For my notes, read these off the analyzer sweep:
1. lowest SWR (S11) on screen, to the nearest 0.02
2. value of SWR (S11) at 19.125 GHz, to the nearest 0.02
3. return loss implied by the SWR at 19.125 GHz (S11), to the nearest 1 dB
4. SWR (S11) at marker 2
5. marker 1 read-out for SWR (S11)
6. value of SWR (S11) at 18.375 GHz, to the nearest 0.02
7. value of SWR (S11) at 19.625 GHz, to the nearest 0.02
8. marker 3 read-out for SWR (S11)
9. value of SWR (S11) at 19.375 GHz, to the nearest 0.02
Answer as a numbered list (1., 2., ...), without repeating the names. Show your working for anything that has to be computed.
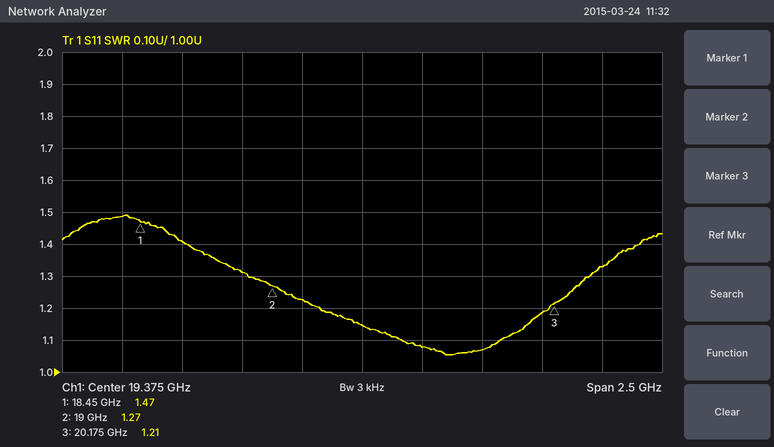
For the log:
1. 1.06
2. 1.22
3. −20 log10((1.22 − 1)/(1.22 + 1)) ≈ 20 dB
4. 1.27
5. 1.47
6. 1.48
7. 1.08
8. 1.21
9. 1.14
